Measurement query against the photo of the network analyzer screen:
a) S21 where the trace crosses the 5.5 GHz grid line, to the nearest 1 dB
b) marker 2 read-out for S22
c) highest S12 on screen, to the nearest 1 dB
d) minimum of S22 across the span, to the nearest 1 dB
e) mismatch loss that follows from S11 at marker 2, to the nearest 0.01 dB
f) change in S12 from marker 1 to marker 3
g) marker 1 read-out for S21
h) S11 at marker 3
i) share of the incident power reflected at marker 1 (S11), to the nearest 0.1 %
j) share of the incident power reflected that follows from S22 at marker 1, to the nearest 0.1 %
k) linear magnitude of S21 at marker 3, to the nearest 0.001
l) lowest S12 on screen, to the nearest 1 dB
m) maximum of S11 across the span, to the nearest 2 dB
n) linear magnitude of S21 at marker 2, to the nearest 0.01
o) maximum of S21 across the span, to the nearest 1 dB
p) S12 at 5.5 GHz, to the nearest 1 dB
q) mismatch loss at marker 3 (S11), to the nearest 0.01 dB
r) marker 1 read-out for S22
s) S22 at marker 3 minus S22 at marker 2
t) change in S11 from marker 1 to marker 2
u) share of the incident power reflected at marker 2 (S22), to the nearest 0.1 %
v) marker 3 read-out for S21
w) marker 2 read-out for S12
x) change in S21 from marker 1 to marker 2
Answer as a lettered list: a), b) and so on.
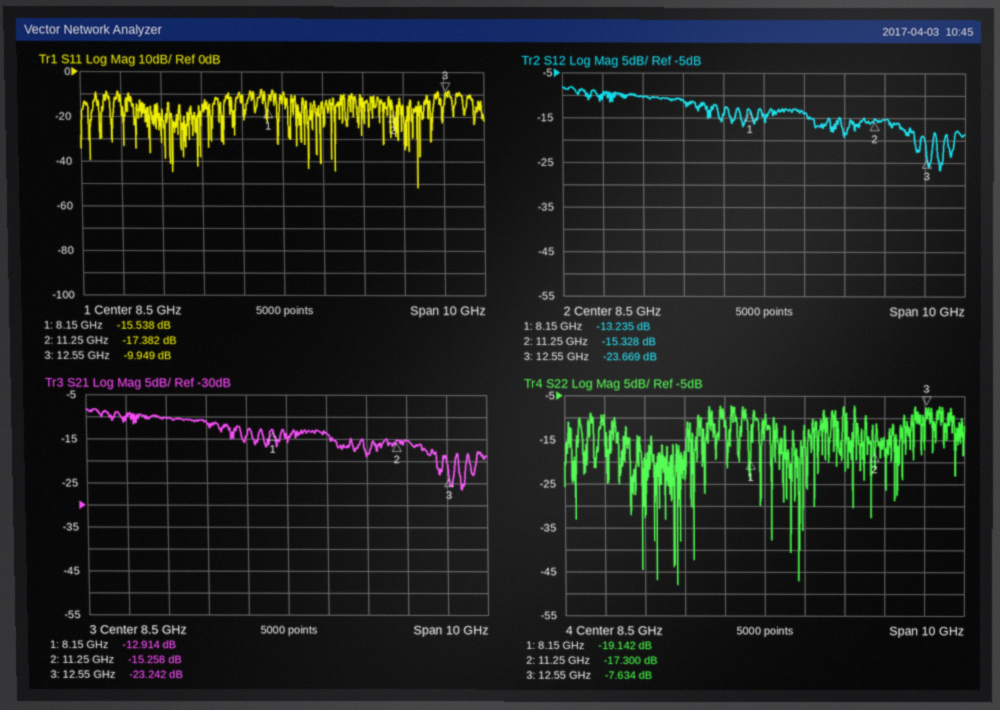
a) -10 dB
b) -17.300 dB
c) -8 dB
d) -48 dB
e) 0.08 dB
f) -10.434 dB
g) -12.914 dB
h) -9.949 dB
i) 2.8 %
j) 1.2 %
k) 0.069
l) -27 dB
m) -8 dB
n) 0.17
o) -8 dB
p) -10 dB
q) 0.46 dB
r) -19.142 dB
s) 9.666 dB
t) -1.844 dB
u) 1.9 %
v) -23.242 dB
w) -15.328 dB
x) -2.344 dB
